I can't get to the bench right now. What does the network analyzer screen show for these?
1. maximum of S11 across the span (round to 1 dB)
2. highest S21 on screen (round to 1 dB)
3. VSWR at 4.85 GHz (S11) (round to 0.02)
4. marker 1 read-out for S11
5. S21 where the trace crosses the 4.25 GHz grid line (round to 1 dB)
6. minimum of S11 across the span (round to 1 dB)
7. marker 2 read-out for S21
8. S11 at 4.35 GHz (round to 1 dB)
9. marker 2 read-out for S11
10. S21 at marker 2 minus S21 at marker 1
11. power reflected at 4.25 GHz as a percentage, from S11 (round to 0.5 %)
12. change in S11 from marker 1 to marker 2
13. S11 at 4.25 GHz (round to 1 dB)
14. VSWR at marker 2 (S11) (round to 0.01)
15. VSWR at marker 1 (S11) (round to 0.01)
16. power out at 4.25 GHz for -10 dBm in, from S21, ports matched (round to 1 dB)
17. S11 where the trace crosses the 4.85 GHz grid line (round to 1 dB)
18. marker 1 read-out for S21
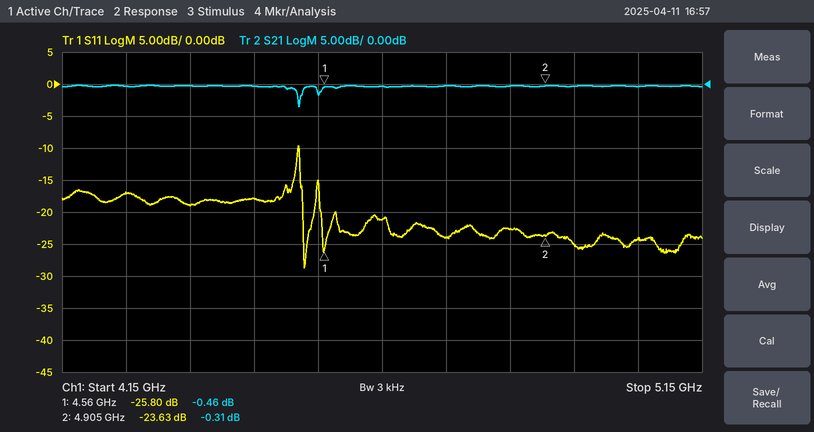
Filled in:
-10 dB
0 dB
1.16
-25.80 dB
0 dB
-29 dB
-0.31 dB
-19 dB
-23.63 dB
0.15 dB
2.0 %
2.17 dB
-17 dB
1.14
1.11
-10 dBm
-23 dB
-0.46 dB
